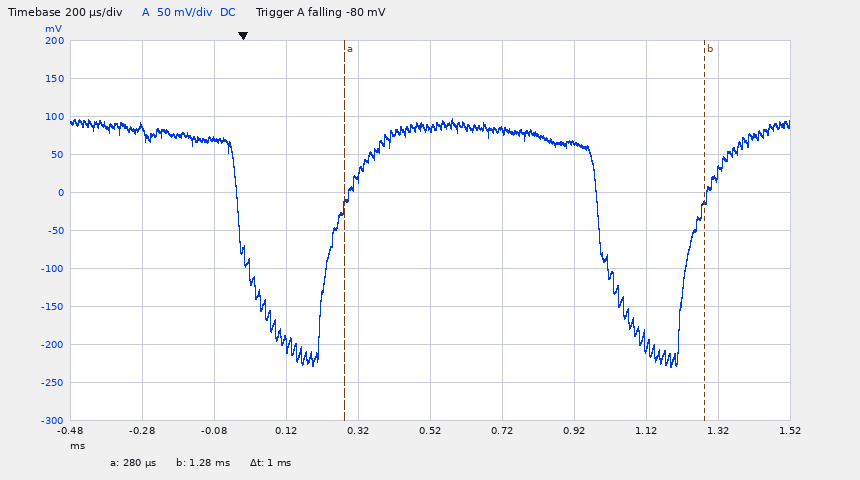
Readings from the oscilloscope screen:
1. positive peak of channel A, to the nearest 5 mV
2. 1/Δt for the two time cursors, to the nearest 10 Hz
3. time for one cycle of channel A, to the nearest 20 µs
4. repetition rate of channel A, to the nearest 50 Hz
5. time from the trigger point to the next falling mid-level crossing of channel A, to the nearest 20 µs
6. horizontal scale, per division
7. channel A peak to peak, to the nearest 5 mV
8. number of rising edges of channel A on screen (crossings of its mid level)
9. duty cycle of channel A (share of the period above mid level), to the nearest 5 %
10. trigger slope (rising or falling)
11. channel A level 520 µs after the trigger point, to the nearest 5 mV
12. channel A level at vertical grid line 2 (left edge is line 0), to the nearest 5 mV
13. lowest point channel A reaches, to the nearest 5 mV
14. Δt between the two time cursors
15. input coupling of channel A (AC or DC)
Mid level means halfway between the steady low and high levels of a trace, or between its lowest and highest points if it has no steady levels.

95 mV
1.00 kHz
1.00 ms
1.00 kHz
1.00 ms
200 µs
325 mV
2
75 %
falling
85 mV
70 mV
-230 mV
1 ms
DC
